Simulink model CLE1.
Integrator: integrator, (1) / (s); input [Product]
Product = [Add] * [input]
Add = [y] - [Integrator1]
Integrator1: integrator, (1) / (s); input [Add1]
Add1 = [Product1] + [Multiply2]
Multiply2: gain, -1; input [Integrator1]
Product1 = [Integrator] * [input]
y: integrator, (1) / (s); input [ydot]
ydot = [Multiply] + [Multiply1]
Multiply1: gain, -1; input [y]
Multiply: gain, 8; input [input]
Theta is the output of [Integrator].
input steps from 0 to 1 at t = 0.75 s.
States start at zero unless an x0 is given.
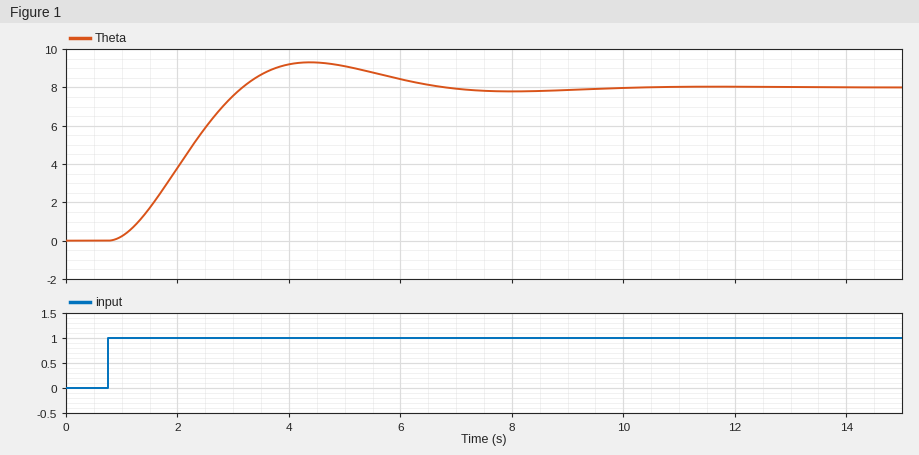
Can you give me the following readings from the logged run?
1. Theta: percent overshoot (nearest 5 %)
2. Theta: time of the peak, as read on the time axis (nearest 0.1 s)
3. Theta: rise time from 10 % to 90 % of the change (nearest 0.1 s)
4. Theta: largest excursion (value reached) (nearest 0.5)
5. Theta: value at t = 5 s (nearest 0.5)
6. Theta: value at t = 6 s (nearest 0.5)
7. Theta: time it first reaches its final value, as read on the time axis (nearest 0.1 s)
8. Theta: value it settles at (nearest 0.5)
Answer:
15 %
4.4 s
1.6 s
9.5
9.0
8.5
3.2 s
8.0
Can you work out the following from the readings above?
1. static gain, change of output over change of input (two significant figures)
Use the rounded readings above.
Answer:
8.0
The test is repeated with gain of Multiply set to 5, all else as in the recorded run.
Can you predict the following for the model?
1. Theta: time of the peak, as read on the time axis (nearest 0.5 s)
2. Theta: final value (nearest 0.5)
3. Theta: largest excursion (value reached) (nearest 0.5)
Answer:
4.5 s
5.0
6.0
